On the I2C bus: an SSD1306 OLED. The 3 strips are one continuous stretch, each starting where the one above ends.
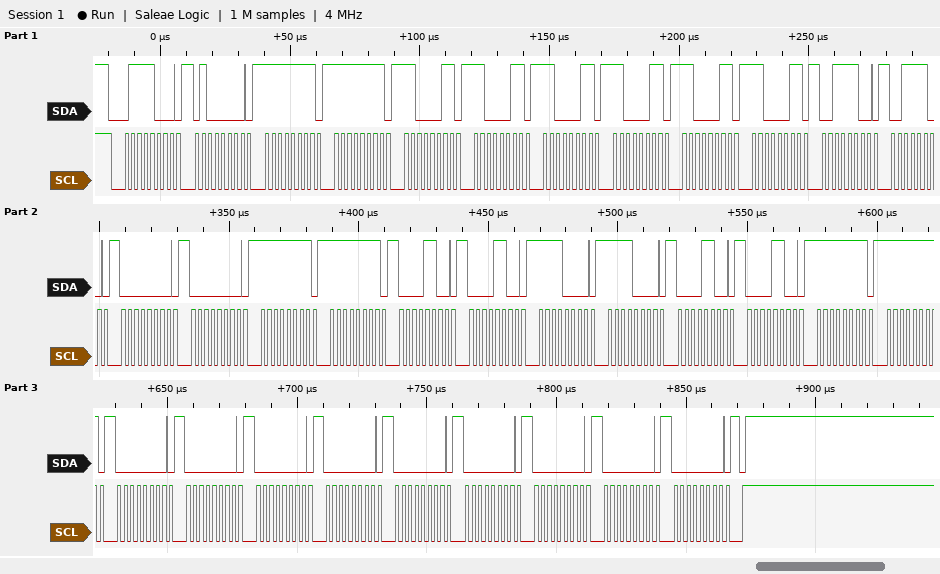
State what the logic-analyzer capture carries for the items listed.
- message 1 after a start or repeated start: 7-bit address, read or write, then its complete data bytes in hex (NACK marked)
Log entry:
0x3C write: 40 FF FF C3 C3 C3 C3 C3 C3 3C 3C 00 00 FF FF 0C 0C F0 F0 0C 0C FF FF 00 00 00 00 00 00 00 00 00
